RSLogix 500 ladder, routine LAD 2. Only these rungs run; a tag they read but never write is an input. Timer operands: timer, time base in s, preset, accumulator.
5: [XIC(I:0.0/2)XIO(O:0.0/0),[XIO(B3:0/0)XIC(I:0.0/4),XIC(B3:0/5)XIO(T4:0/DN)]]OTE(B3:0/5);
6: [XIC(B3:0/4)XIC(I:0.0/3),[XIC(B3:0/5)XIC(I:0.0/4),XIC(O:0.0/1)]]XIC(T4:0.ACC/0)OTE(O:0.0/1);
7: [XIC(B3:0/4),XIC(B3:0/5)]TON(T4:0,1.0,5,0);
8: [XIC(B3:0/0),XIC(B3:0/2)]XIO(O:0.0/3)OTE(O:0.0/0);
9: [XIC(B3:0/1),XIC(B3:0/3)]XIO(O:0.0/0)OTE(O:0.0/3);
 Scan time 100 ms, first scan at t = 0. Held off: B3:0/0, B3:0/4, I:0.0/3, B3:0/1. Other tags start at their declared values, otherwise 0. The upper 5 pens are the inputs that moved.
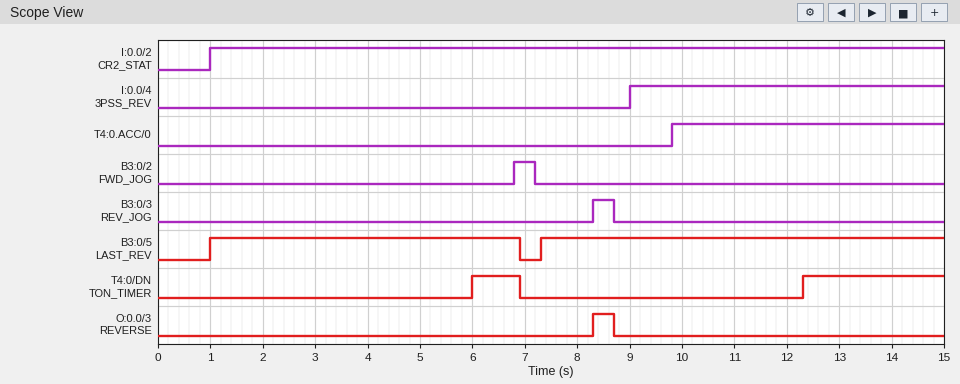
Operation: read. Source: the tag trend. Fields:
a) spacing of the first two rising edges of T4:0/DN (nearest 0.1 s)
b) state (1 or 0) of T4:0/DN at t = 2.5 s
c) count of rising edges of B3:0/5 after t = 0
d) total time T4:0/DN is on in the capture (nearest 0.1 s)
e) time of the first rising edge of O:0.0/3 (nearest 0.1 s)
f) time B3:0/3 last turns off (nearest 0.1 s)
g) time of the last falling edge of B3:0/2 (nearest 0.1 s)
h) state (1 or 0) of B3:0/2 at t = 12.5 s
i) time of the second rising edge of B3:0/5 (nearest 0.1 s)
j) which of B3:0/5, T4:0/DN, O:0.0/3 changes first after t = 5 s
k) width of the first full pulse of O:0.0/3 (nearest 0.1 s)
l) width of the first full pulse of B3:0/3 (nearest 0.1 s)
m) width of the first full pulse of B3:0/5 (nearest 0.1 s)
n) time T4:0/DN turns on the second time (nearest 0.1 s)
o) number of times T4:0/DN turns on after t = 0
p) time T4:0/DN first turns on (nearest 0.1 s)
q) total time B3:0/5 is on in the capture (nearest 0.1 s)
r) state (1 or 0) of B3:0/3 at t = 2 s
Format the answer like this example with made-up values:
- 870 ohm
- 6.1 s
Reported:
- 6.3 s
- 0
- 2
- 3.6 s
- 8.3 s
- 8.7 s
- 7.2 s
- 0
- 7.3 s
- T4:0/DN
- 0.4 s
- 0.4 s
- 5.9 s
- 12.3 s
- 2
- 6.0 s
- 13.6 s
- 0
